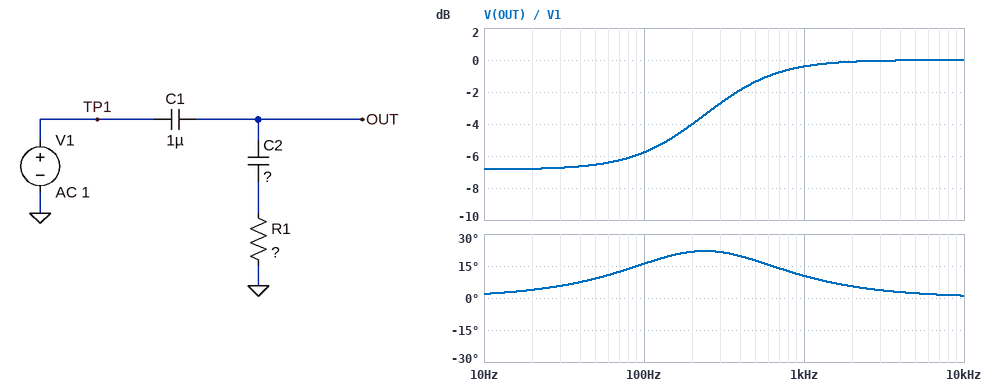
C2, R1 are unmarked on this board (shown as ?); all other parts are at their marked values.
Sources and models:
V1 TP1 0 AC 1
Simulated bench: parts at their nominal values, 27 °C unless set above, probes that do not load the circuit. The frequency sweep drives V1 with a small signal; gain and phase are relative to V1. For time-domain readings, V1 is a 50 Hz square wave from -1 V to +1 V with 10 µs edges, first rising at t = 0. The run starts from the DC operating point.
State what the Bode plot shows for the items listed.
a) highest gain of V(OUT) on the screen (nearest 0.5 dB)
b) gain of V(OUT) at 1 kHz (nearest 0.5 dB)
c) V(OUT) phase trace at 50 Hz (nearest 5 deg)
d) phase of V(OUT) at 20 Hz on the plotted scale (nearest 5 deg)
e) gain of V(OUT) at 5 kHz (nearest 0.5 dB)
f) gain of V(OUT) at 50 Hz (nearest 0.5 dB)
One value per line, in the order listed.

0 dB
-0.5 dB
10 deg
5 deg
0 dB
-6.5 dB
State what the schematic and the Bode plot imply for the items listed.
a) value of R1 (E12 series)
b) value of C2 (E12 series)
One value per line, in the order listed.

820 Ω
1.2 µF
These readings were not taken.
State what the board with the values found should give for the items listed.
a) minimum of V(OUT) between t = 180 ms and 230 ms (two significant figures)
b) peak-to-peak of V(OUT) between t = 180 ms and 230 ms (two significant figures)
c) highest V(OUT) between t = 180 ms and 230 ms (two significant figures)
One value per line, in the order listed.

-1.1 V
3.1 V
2.0 V
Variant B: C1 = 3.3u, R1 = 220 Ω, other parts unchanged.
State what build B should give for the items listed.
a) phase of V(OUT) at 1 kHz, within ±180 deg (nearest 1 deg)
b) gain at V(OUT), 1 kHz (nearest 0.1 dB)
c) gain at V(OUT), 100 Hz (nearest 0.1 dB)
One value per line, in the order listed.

8 deg
-0.9 dB
-2.6 dB
